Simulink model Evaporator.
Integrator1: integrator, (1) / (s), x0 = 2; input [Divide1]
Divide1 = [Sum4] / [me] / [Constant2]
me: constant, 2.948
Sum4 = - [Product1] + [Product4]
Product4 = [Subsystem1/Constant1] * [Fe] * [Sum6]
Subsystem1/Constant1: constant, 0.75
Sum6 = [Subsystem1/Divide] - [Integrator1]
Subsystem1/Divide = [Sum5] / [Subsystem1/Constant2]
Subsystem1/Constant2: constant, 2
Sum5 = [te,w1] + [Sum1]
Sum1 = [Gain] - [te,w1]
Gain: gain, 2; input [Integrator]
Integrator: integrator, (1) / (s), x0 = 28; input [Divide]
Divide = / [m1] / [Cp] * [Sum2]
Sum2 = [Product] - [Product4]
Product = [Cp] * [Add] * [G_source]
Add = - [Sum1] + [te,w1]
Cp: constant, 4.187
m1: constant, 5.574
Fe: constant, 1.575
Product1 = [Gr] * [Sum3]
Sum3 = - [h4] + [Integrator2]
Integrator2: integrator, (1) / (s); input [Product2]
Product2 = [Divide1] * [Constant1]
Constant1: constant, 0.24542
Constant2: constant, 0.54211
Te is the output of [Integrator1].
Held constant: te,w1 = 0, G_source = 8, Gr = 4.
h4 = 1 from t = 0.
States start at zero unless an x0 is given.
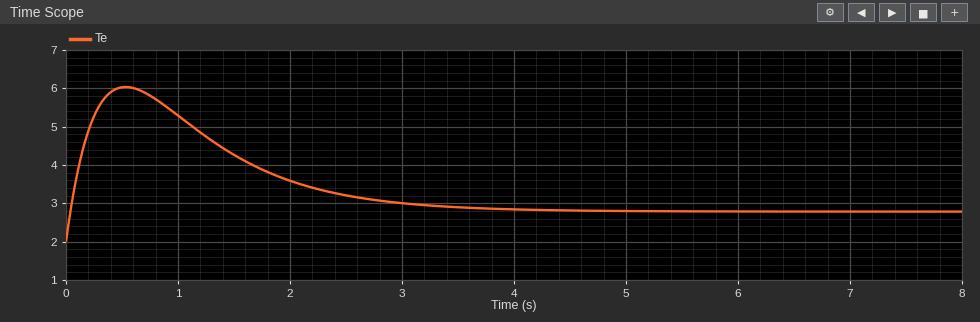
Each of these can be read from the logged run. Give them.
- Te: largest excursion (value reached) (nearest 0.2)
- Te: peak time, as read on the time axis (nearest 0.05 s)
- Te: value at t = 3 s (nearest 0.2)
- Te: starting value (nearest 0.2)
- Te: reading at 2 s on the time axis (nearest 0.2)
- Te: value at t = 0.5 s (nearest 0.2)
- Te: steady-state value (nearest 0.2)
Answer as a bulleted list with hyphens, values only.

- 6.0
- 0.55 s
- 3.0
- 2.0
- 3.6
- 6.0
- 2.8
